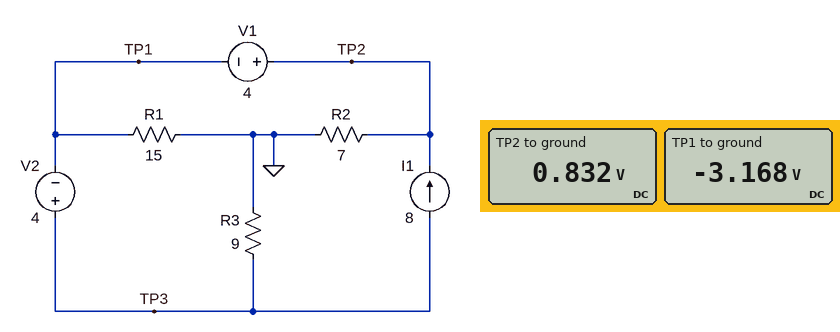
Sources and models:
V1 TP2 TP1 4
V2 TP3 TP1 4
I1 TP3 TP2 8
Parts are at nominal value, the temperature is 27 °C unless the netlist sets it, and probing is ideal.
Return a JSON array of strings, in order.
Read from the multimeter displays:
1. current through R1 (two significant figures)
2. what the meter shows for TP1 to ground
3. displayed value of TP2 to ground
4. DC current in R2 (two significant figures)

["210 mA", "-3.168 V", "0.832 V", "120 mA"]
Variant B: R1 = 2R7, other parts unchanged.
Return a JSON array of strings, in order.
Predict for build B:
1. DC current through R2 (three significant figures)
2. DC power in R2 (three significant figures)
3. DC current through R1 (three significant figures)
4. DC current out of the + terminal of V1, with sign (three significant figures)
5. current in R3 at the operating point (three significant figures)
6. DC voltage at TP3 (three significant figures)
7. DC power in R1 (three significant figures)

["339 mA", "804 mW", "603 mA", "-7.66 A", "264 mA", "2.37 V", "981 mW"]
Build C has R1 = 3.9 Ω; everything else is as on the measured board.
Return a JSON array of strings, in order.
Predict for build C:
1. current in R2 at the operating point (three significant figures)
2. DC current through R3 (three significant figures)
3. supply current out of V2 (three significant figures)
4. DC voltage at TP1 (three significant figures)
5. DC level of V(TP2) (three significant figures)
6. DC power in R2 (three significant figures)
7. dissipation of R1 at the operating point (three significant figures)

["287 mA", "223 mA", "8.22 A", "-1.99 V", "2.01 V", "577 mW", "1.02 W"]
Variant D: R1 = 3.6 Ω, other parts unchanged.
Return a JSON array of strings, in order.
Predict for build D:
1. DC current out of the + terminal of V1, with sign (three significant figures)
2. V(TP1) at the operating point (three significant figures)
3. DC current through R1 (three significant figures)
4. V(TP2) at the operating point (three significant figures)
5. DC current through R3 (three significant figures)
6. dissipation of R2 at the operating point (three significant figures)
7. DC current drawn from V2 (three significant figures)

["-7.70 A", "-1.91 V", "531 mA", "2.09 V", "232 mA", "624 mW", "8.23 A"]
